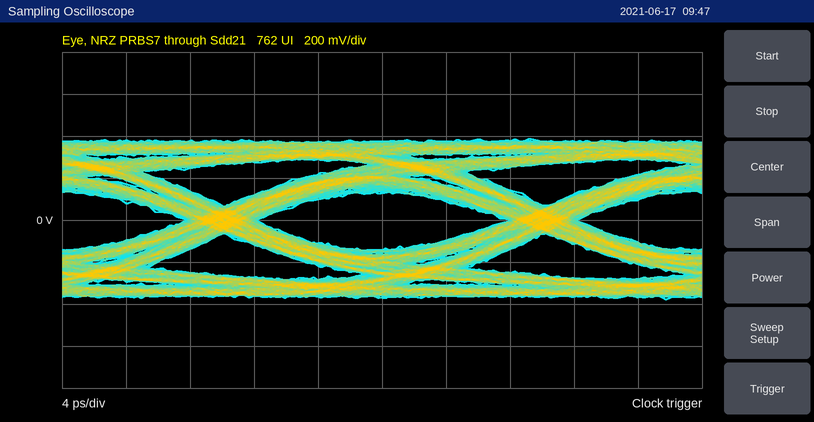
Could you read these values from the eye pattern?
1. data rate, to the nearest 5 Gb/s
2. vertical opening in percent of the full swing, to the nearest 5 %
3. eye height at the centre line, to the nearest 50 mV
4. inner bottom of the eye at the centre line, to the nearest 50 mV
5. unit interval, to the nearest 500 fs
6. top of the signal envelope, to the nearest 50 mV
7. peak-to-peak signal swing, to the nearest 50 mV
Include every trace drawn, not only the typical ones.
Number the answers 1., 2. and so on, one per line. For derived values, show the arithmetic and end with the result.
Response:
1. 50 Gb/s
2. 250 mV / 750 mV ≈ 33.3 %, so 35 % to the nearest 5 %
3. 250 mV
4. -150 mV
5. 20.0 ps
6. 400 mV
7. 750 mV
